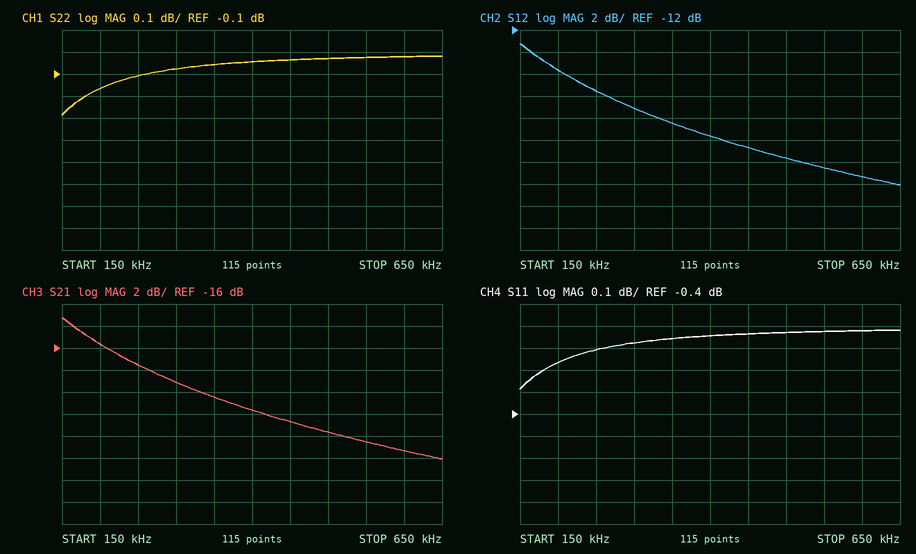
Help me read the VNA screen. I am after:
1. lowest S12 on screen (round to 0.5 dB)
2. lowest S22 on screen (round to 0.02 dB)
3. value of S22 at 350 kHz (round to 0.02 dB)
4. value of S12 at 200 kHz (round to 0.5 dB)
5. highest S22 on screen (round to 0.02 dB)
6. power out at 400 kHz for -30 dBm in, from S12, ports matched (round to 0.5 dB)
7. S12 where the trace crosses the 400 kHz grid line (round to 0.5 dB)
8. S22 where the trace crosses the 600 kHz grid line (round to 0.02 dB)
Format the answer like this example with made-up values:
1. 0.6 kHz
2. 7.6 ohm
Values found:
1. -26.0 dB
2. -0.28 dB
3. -0.06 dB
4. -15.5 dB
5. -0.02 dB
6. -51.5 dBm
7. -21.5 dB
8. -0.02 dB
